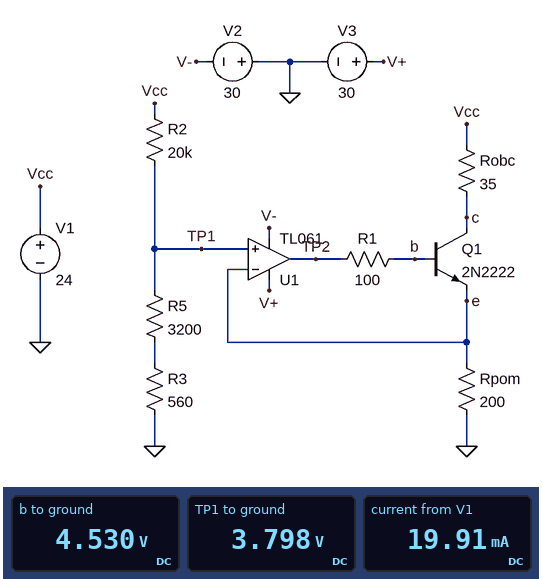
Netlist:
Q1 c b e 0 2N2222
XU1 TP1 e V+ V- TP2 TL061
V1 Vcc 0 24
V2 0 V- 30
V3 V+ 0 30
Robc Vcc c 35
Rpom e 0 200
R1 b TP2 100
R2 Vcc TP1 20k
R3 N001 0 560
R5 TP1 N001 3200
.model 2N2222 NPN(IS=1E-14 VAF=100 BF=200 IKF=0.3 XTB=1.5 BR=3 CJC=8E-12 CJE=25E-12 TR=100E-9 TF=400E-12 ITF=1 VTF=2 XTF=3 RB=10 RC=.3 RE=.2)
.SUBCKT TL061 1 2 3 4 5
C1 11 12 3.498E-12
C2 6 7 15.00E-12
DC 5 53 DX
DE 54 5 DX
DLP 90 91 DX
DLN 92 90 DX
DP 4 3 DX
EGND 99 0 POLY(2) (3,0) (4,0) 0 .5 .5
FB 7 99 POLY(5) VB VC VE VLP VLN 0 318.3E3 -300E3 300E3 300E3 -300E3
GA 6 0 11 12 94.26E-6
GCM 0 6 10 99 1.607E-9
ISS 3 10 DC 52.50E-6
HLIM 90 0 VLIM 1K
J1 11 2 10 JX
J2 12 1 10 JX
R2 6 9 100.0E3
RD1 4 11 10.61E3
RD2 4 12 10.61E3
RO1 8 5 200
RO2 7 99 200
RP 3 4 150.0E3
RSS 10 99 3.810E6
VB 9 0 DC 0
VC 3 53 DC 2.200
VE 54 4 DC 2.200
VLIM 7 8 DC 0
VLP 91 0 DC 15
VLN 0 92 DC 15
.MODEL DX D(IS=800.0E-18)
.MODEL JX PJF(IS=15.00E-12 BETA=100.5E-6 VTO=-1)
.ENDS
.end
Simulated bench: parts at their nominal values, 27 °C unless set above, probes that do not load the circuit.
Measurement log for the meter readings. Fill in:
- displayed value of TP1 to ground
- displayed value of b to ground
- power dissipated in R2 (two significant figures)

3.798 V
4.530 V
20 mW
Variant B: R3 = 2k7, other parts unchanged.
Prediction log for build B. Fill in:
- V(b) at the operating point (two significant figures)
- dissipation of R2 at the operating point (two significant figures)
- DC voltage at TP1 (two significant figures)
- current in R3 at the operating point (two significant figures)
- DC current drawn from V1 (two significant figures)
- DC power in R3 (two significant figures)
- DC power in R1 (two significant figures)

6.2 V
17 mW
5.5 V
930 µA
28 mA
2.3 mW
1.6 µW
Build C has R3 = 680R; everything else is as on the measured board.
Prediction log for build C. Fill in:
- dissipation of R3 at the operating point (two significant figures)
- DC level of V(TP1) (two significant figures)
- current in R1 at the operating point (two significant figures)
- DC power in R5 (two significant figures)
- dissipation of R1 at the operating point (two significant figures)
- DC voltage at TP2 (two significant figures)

690 µW
3.9 V
86 µA
3.2 mW
740 nW
4.6 V
